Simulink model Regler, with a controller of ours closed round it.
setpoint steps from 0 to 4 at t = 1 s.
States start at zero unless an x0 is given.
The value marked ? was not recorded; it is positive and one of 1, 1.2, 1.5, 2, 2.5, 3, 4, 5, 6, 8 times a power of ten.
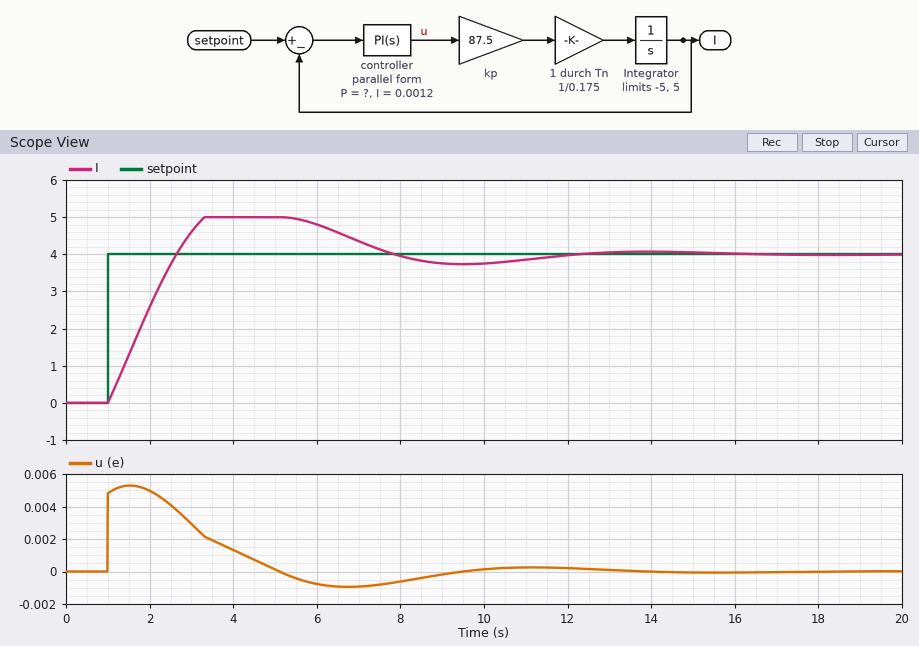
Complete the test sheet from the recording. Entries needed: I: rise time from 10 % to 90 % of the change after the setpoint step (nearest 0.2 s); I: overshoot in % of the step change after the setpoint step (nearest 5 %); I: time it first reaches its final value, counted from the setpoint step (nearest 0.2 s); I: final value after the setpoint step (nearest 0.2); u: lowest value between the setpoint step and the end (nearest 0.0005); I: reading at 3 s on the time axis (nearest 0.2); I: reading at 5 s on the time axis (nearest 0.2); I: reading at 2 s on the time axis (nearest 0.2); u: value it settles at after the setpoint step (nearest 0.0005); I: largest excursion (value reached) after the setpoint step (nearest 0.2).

1.2 s
25 %
1.6 s
4.0
-0.0010
4.6
5.0
2.6
0.0000
5.0
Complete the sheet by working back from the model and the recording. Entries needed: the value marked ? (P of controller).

0.0012
